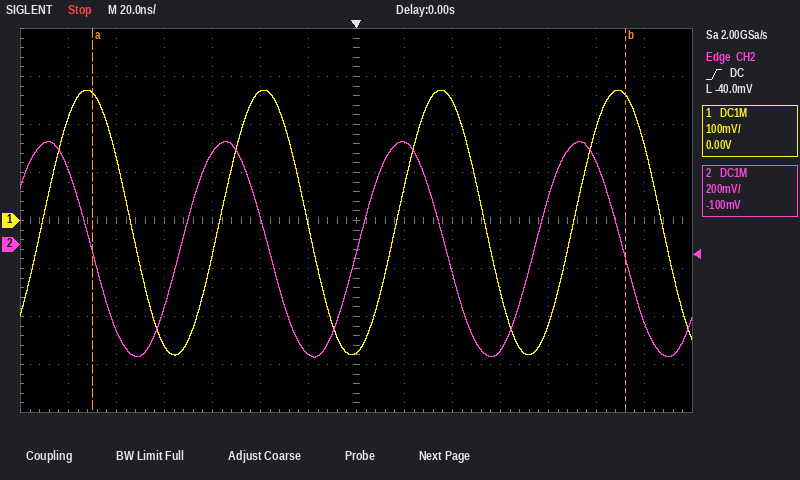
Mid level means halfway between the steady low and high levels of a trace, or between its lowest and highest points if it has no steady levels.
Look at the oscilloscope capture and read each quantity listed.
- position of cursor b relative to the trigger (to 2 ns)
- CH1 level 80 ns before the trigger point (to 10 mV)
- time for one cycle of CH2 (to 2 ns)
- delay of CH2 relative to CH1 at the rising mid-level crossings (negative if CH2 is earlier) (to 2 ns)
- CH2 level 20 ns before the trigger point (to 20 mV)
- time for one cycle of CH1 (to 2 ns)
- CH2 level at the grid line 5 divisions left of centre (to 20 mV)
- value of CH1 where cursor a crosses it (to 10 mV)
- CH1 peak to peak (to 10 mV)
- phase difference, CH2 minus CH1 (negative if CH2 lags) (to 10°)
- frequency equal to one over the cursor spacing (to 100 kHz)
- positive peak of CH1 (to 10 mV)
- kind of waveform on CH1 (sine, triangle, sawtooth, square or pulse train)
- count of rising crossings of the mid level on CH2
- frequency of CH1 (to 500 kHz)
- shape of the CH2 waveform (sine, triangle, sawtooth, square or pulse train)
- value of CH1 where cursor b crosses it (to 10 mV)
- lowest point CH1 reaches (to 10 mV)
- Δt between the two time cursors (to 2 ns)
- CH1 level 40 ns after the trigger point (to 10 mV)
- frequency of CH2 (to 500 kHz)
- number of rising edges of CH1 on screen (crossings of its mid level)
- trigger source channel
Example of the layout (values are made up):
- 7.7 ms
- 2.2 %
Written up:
- +112 ns
- -260 mV
- 74 ns
- -16 ns
- -460 mV
- 74 ns
- -360 mV
- 260 mV
- 550 mV
- +80°
- 4.5 MHz
- 270 mV
- sine
- 3
- 13.5 MHz
- sine
- 260 mV
- -280 mV
- 222 ns
- 250 mV
- 13.5 MHz
- 4
- CH2
